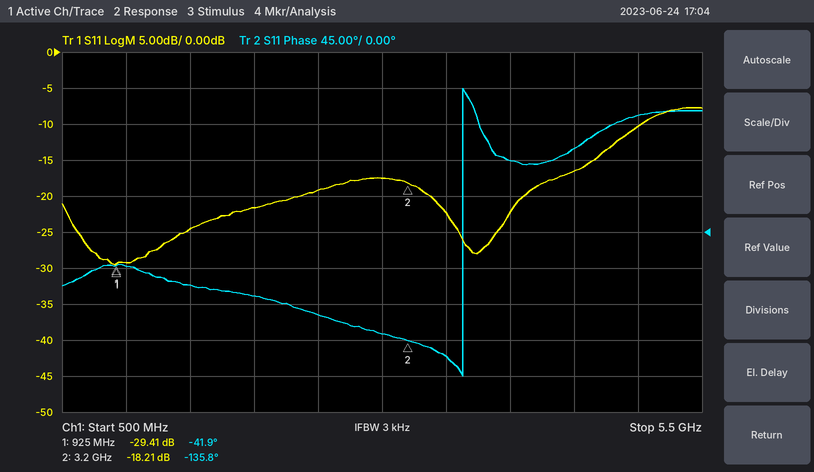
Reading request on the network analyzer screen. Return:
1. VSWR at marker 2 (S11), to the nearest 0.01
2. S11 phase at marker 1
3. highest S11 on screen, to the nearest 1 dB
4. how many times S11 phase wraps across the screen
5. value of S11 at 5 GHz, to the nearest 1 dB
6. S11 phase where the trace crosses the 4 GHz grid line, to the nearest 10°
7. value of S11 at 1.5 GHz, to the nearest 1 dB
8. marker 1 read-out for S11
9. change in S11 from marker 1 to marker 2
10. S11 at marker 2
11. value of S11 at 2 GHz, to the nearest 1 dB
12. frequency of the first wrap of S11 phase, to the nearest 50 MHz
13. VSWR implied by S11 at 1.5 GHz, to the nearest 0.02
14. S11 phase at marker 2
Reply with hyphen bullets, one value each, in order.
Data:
- 1.28
- -41.9°
- -8 dB
- 1
- -10 dB
- 90°
- -25 dB
- -29.41 dB
- 11.20 dB
- -18.21 dB
- -22 dB
- 3.65 GHz
- 1.12
- -135.8°
